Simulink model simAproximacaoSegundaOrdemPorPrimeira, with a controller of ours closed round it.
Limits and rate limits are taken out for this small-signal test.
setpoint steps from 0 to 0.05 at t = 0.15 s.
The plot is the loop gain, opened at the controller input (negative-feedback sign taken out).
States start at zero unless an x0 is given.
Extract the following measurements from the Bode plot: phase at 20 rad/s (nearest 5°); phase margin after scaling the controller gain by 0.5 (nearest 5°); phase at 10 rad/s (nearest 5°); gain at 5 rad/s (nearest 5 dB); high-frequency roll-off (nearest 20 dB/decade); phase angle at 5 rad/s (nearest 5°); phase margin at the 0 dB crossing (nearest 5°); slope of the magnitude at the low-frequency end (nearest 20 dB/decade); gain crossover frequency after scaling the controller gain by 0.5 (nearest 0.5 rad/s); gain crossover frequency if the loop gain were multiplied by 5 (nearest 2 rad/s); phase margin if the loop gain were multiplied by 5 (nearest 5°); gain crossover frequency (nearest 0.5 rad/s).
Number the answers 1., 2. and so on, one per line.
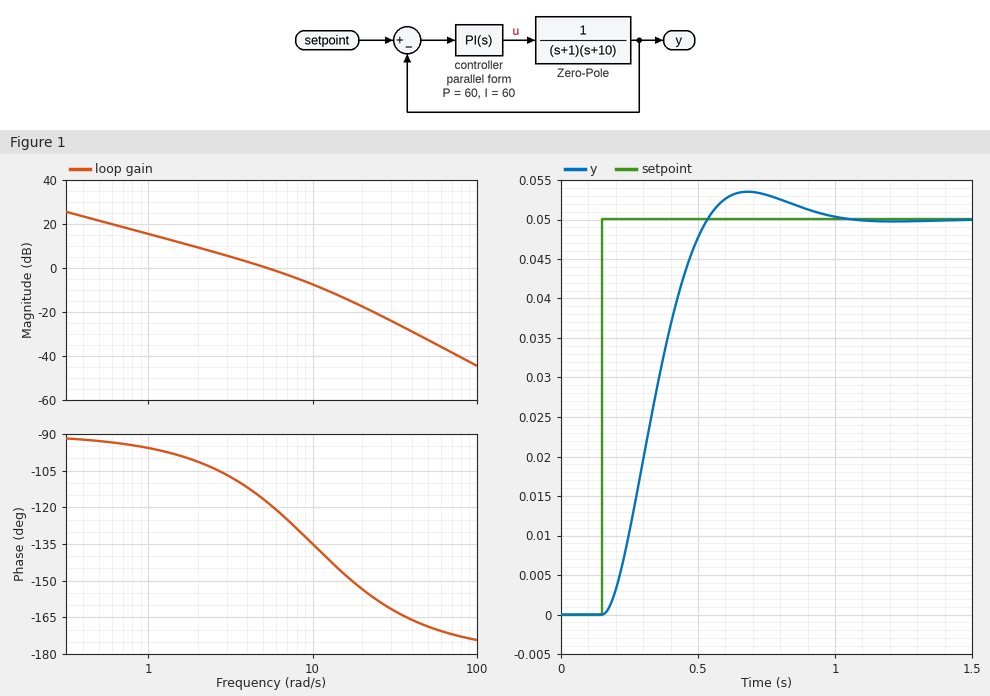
1. -155°
2. 75°
3. -135°
4. 0 dB
5. -40 dB/decade
6. -115°
7. 60°
8. -20 dB/decade
9. 3.0 rad/s
10. 16 rad/s
11. 30°
12. 5.5 rad/s
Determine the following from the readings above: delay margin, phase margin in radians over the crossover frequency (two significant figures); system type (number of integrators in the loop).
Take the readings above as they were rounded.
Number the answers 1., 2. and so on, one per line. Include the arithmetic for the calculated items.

1. 60 × π / 180 / 5.5 = 0.19 s
2. 1
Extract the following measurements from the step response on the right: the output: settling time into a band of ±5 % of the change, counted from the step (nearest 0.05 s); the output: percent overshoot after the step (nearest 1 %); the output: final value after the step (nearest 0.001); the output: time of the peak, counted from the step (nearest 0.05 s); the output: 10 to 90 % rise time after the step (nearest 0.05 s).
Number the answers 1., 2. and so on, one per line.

1. 0.65 s
2. 7 %
3. 0.050
4. 0.55 s
5. 0.25 s
